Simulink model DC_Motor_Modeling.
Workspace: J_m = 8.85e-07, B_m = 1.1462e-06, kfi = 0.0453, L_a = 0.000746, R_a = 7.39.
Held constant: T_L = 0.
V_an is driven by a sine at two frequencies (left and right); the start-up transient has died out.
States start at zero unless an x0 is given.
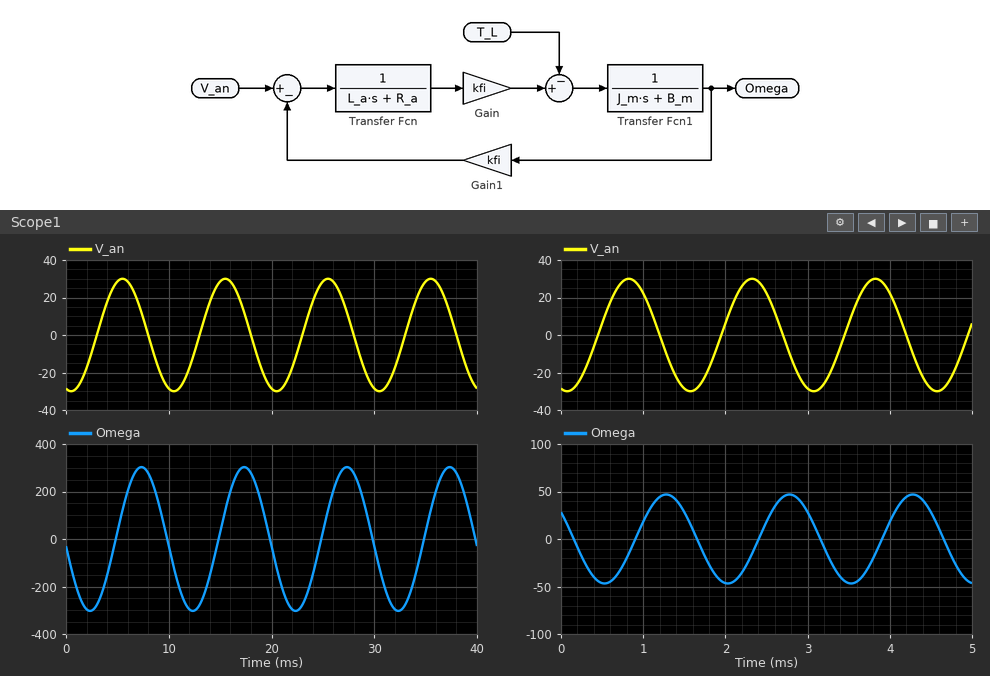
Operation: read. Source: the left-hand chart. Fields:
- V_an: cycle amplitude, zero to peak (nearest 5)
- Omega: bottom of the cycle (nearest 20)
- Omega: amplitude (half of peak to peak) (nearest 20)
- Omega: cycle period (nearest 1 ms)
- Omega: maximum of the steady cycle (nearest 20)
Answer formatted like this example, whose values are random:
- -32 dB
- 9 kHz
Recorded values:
- 30
- -300
- 300
- 10 ms
- 300
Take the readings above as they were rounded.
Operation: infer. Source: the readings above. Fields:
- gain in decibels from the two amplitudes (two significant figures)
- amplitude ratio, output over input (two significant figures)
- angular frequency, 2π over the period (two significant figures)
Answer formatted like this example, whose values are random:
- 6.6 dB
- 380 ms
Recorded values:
- 20 dB
- 10
- 0.63 rad/ms
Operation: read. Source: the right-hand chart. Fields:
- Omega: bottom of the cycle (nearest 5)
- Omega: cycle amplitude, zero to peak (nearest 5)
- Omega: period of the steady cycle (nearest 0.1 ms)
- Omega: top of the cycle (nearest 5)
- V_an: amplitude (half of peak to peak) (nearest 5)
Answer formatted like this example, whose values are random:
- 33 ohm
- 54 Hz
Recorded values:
- -45
- 45
- 1.5 ms
- 45
- 30
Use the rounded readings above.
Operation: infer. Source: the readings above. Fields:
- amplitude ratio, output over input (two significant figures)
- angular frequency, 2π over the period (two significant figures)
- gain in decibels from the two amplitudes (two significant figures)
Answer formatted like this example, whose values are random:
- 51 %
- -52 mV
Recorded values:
- 1.5
- 4.2 rad/ms
- 3.5 dB
